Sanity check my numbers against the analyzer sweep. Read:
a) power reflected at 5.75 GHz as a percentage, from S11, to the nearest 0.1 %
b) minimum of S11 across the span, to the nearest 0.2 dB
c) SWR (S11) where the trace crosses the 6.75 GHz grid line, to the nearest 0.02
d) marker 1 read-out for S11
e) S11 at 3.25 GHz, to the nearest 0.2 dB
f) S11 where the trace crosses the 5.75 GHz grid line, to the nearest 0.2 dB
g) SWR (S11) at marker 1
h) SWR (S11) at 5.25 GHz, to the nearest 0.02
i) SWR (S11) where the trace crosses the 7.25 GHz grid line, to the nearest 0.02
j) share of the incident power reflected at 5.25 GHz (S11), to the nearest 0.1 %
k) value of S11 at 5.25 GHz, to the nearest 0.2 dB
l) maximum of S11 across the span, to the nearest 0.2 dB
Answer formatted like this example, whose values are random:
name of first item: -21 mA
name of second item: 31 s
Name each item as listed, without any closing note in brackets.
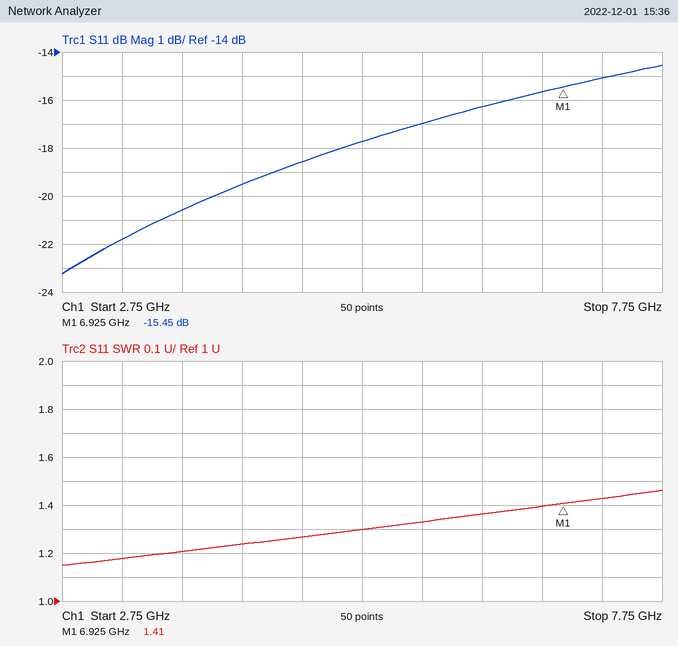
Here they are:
power reflected at 5.75 GHz as a percentage, from S11, to the nearest 0.1 %: 2.0 %
minimum of S11 across the span, to the nearest 0.2 dB: -23.2 dB
SWR (S11) where the trace crosses the 6.75 GHz grid line, to the nearest 0.02: 1.40
marker 1 read-out for S11: -15.45 dB
S11 at 3.25 GHz, to the nearest 0.2 dB: -21.8 dB
S11 where the trace crosses the 5.75 GHz grid line, to the nearest 0.2 dB: -17.0 dB
SWR (S11) at marker 1: 1.41
SWR (S11) at 5.25 GHz, to the nearest 0.02: 1.30
SWR (S11) where the trace crosses the 7.25 GHz grid line, to the nearest 0.02: 1.42
share of the incident power reflected at 5.25 GHz (S11), to the nearest 0.1 %: 1.7 %
value of S11 at 5.25 GHz, to the nearest 0.2 dB: -17.8 dB
maximum of S11 across the span, to the nearest 0.2 dB: -14.6 dB
